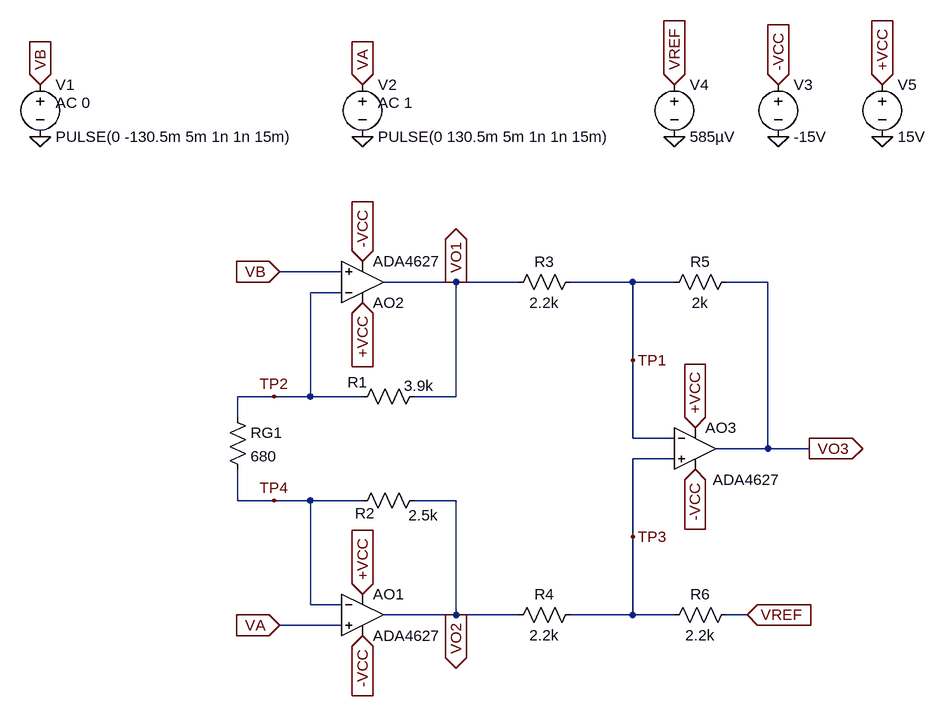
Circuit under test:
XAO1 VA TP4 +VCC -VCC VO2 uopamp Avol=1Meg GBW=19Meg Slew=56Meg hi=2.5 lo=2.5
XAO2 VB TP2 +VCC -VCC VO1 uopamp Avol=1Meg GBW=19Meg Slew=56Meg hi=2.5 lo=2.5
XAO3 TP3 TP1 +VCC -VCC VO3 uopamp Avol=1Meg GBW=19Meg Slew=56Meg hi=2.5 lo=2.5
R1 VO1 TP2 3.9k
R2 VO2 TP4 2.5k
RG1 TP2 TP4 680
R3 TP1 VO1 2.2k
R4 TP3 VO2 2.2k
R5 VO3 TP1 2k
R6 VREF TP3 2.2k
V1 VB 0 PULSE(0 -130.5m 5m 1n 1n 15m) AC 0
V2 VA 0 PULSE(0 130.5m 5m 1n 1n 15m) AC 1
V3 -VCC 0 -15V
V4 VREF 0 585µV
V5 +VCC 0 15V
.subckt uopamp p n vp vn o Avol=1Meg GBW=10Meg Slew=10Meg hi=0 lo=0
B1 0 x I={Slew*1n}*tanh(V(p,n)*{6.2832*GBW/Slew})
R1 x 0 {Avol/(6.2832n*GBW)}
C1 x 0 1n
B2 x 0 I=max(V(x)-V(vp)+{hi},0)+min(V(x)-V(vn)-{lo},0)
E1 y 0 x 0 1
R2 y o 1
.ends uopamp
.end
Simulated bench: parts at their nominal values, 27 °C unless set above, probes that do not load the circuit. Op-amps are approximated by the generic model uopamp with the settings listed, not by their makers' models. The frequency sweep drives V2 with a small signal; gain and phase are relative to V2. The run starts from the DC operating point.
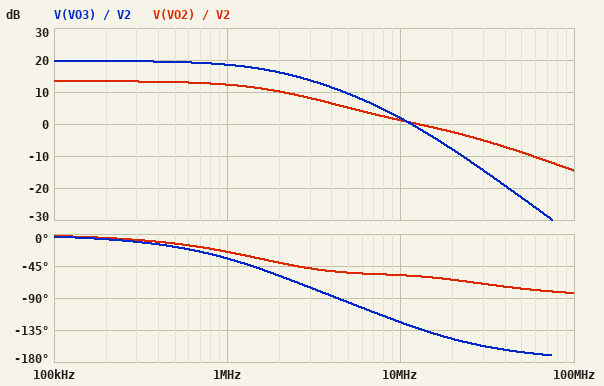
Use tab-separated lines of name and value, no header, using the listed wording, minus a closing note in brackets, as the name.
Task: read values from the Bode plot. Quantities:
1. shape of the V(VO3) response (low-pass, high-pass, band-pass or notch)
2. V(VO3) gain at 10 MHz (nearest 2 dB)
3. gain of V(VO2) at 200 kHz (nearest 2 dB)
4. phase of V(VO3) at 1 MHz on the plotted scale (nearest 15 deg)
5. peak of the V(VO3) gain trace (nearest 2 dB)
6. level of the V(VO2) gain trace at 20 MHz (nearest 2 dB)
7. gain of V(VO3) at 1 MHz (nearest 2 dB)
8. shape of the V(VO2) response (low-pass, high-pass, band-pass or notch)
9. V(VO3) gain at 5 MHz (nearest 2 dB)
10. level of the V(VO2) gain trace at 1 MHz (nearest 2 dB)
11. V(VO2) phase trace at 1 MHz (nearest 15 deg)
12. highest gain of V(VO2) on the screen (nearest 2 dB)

shape of the V(VO3) response	low-pass
V(VO3) gain at 10 MHz	2 dB
gain of V(VO2) at 200 kHz	14 dB
phase of V(VO3) at 1 MHz on the plotted scale	-30 deg
peak of the V(VO3) gain trace	20 dB
level of the V(VO2) gain trace at 20 MHz	-2 dB
gain of V(VO3) at 1 MHz	18 dB
shape of the V(VO2) response	low-pass
V(VO3) gain at 5 MHz	10 dB
level of the V(VO2) gain trace at 1 MHz	12 dB
V(VO2) phase trace at 1 MHz	-30 deg
highest gain of V(VO2) on the screen	14 dB
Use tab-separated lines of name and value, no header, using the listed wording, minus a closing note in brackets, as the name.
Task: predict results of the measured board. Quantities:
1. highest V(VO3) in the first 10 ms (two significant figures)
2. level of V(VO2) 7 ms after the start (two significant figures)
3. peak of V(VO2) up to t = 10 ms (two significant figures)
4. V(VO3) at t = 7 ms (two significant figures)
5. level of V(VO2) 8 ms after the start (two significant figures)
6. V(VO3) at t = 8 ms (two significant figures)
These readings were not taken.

highest V(VO3) in the first 10 ms	2.5 V
level of V(VO2) 7 ms after the start	1.1 V
peak of V(VO2) up to t = 10 ms	1.1 V
V(VO3) at t = 7 ms	2.5 V
level of V(VO2) 8 ms after the start	1.1 V
V(VO3) at t = 8 ms	2.5 V
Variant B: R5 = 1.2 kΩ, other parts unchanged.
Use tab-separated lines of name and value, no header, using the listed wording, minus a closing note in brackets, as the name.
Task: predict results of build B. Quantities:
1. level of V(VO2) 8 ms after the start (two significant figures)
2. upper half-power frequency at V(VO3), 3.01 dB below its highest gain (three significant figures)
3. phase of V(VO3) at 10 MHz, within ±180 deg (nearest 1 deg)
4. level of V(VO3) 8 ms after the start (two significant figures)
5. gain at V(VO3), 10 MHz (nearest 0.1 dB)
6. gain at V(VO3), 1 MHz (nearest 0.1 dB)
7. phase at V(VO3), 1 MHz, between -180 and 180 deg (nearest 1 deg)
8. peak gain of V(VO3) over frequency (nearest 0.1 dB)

level of V(VO2) 8 ms after the start	1.1 V
upper half-power frequency at V(VO3), 3.01 dB below its highest gain	1.79 MHz
phase of V(VO3) at 10 MHz, within ±180 deg	-114 deg
level of V(VO3) 8 ms after the start	1.7 V
gain at V(VO3), 10 MHz	-0.2 dB
gain at V(VO3), 1 MHz	15.4 dB
phase at V(VO3), 1 MHz, between -180 and 180 deg	-33 deg
peak gain of V(VO3) over frequency	16.6 dB
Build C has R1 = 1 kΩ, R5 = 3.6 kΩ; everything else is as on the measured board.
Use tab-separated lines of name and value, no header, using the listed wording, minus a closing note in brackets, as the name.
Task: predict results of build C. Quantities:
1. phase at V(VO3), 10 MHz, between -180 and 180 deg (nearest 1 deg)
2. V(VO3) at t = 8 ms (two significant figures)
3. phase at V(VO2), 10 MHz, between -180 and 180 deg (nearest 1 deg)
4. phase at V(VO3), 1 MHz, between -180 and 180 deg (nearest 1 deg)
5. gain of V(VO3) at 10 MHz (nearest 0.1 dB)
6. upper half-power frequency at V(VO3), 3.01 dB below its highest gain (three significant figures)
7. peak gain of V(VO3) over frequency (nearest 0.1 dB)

phase at V(VO3), 10 MHz, between -180 and 180 deg	-128 deg
V(VO3) at t = 8 ms	2.3 V
phase at V(VO2), 10 MHz, between -180 and 180 deg	-66 deg
phase at V(VO3), 1 MHz, between -180 and 180 deg	-26 deg
gain of V(VO3) at 10 MHz	3.3 dB
upper half-power frequency at V(VO3), 3.01 dB below its highest gain	2.68 MHz
peak gain of V(VO3) over frequency	18.7 dB
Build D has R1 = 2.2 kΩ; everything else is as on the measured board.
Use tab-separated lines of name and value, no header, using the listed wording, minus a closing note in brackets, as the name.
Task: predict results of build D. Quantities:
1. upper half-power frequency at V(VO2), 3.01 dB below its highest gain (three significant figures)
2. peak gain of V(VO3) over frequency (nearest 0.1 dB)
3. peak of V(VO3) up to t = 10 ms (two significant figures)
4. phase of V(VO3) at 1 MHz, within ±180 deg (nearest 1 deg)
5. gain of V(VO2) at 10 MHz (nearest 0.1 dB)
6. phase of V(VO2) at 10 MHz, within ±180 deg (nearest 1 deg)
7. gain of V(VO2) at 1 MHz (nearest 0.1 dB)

upper half-power frequency at V(VO2), 3.01 dB below its highest gain	2.47 MHz
peak gain of V(VO3) over frequency	17.4 dB
peak of V(VO3) up to t = 10 ms	1.9 V
phase of V(VO3) at 1 MHz, within ±180 deg	-28 deg
gain of V(VO2) at 10 MHz	2.2 dB
phase of V(VO2) at 10 MHz, within ±180 deg	-63 deg
gain of V(VO2) at 1 MHz	12.7 dB
